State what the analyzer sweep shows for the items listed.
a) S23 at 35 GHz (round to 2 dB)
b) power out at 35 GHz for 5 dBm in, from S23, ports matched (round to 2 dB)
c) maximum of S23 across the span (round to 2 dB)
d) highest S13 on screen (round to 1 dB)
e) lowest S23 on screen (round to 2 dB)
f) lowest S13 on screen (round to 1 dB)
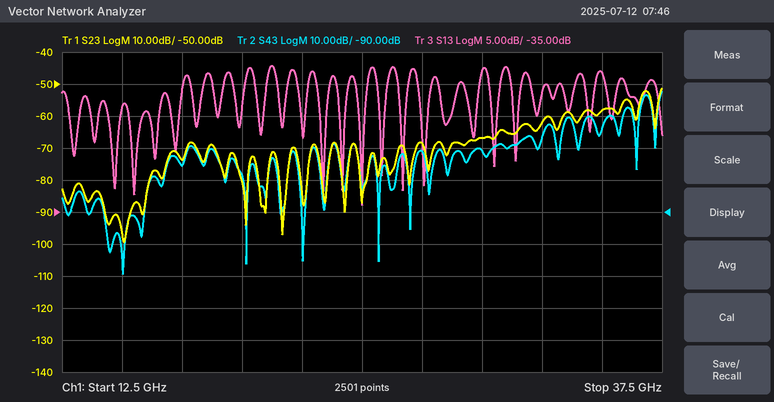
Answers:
-58 dB
-54 dBm
-52 dB
-12 dB
-100 dB
-34 dB
